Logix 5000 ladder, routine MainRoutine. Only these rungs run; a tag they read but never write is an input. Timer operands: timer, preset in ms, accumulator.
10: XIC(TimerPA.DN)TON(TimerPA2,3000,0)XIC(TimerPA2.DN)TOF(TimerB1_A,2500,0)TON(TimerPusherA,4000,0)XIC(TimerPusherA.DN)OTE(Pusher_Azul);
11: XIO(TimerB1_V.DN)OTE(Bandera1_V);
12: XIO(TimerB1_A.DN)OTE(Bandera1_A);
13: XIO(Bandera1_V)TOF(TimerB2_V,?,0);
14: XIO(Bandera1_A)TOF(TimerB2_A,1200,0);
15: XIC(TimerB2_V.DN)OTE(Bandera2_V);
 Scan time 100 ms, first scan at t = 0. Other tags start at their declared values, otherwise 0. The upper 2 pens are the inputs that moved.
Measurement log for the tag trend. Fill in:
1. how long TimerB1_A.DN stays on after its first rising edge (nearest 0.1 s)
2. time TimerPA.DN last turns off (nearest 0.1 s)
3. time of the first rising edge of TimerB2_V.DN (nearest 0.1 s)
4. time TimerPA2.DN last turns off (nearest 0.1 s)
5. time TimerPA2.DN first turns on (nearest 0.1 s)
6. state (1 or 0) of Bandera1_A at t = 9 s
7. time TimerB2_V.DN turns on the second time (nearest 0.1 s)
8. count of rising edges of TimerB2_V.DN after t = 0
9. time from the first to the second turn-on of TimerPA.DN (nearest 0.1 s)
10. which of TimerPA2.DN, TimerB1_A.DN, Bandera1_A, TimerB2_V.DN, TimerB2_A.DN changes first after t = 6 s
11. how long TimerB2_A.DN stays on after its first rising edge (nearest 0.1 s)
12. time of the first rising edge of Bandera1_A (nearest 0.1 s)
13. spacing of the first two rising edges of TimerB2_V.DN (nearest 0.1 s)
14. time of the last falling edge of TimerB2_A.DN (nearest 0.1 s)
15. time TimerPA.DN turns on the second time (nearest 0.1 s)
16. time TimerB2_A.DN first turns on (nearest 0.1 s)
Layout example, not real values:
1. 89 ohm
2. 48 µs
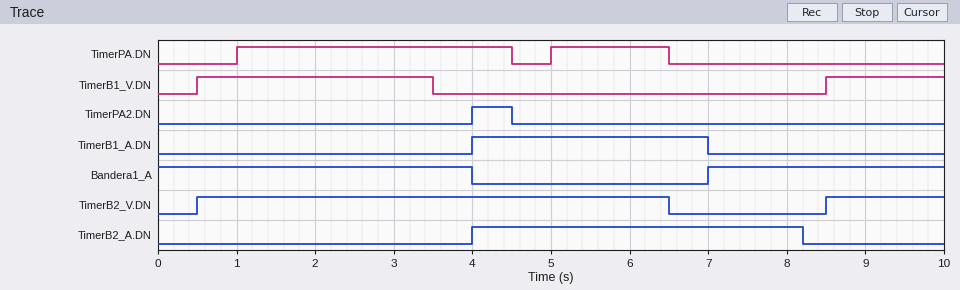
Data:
1. 3.0 s
2. 6.5 s
3. 0.5 s
4. 4.5 s
5. 4.0 s
6. 1
7. 8.5 s
8. 2
9. 4.0 s
10. TimerB2_V.DN
11. 4.2 s
12. 7.0 s
13. 8.0 s
14. 8.2 s
15. 5.0 s
16. 4.0 s
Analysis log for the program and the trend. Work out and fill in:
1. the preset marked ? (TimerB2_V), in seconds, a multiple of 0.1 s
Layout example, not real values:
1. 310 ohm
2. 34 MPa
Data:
1. 3.0 s
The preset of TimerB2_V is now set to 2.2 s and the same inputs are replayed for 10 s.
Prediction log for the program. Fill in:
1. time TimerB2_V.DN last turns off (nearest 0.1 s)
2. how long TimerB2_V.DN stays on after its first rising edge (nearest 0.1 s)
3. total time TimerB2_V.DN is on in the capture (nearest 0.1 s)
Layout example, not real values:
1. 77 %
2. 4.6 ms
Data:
1. 5.7 s
2. 5.2 s
3. 6.7 s
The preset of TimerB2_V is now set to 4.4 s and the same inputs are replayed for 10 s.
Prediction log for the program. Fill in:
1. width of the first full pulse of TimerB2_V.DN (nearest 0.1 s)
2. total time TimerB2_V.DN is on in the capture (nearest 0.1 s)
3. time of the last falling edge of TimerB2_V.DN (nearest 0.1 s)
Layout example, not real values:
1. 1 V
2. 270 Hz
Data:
1. 7.4 s
2. 8.9 s
3. 7.9 s
